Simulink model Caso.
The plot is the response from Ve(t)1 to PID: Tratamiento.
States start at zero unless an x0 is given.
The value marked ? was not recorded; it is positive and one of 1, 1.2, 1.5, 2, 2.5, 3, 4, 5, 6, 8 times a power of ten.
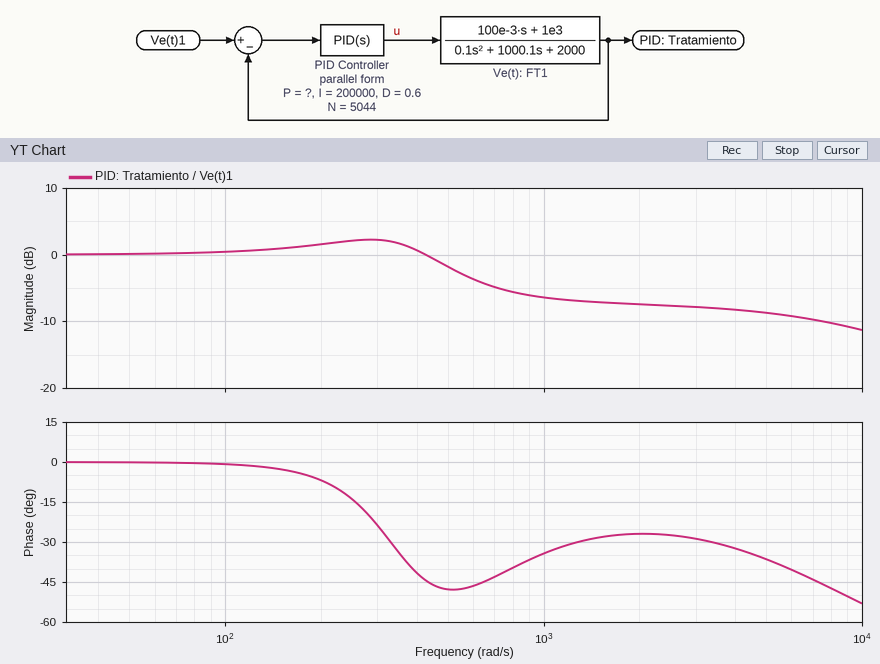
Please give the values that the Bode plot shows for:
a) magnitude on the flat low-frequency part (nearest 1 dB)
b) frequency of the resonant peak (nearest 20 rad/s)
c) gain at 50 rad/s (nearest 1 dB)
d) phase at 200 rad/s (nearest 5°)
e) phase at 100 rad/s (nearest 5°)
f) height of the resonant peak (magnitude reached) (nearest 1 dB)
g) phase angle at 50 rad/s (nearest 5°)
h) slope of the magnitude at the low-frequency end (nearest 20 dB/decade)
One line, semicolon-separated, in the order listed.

0 dB; 280 rad/s; 0 dB; -5°; 0°; 2 dB; 0°; 0 dB/decade
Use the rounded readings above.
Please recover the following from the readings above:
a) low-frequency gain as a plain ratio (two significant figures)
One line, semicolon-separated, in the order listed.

1.0
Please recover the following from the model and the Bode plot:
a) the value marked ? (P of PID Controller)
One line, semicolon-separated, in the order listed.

500
